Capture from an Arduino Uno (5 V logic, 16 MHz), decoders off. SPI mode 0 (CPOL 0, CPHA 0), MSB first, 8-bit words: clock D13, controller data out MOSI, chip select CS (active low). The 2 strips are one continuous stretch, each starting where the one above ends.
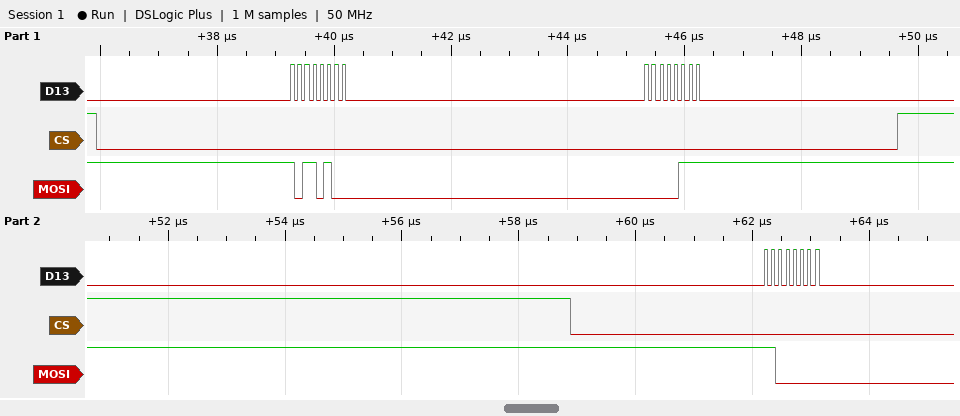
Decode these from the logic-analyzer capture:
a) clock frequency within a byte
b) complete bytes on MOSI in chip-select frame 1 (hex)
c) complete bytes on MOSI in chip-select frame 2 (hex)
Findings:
8 MHz
B4 07
C0
